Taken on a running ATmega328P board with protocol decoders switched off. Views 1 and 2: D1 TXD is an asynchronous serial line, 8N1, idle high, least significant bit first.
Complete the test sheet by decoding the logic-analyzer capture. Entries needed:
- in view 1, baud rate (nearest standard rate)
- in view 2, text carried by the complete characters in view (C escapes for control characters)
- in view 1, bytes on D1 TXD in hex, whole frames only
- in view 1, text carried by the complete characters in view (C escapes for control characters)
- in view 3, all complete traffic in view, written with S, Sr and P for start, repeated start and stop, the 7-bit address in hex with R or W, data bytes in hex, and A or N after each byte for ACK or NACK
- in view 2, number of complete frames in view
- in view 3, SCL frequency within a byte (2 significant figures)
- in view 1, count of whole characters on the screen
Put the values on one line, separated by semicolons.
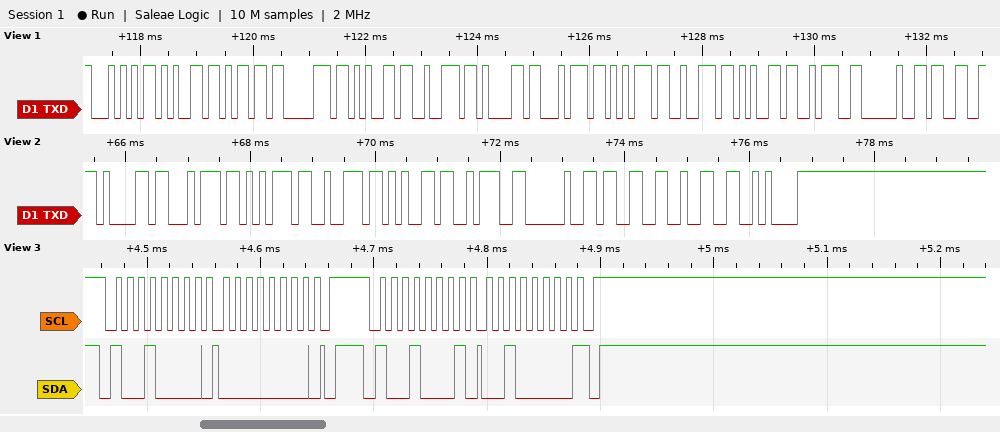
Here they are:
9600 baud; "ature: 32\n"; 54 65 6D 70 65 72 61 74 75 72 65 3A 20 33; "Temperature: 3"; S 48W A 00 A P S 48R A 20 N P; 10; 100 kHz; 14
